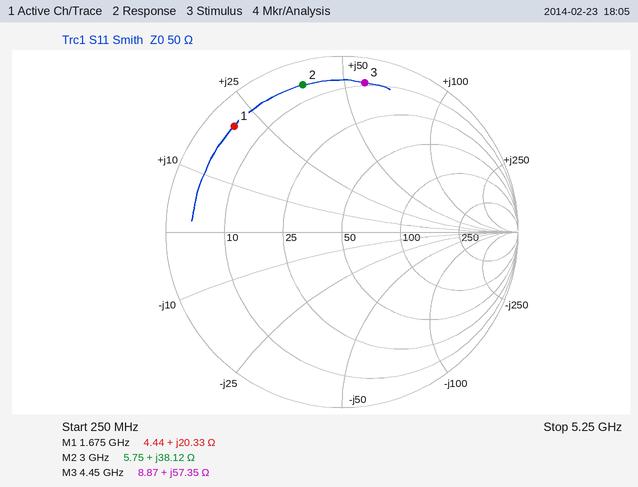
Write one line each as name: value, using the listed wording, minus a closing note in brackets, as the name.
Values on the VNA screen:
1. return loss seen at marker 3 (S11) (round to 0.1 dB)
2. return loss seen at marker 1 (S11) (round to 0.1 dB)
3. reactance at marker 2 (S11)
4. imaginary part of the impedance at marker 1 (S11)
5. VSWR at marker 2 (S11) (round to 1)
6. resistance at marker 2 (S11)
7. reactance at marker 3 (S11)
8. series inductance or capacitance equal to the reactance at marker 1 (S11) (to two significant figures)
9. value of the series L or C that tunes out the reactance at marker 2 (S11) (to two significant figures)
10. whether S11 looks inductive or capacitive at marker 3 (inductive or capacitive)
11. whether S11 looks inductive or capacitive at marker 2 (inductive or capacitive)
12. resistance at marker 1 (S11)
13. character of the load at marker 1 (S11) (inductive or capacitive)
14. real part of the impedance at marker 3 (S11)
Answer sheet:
return loss seen at marker 3 (S11): 1.3 dB
return loss seen at marker 1 (S11): 1.3 dB
reactance at marker 2: +38.12 Ω
imaginary part of the impedance at marker 1: +20.33 Ω
VSWR at marker 2 (S11): 14
resistance at marker 2: 5.75 Ω
reactance at marker 3: +57.35 Ω
series inductance or capacitance equal to the reactance at marker 1 (S11): 1.9 nH
value of the series L or C that tunes out the reactance at marker 2 (S11): 1.4 pF
whether S11 looks inductive or capacitive at marker 3: inductive
whether S11 looks inductive or capacitive at marker 2: inductive
resistance at marker 1: 4.44 Ω
character of the load at marker 1 (S11): inductive
real part of the impedance at marker 3: 8.87 Ω
